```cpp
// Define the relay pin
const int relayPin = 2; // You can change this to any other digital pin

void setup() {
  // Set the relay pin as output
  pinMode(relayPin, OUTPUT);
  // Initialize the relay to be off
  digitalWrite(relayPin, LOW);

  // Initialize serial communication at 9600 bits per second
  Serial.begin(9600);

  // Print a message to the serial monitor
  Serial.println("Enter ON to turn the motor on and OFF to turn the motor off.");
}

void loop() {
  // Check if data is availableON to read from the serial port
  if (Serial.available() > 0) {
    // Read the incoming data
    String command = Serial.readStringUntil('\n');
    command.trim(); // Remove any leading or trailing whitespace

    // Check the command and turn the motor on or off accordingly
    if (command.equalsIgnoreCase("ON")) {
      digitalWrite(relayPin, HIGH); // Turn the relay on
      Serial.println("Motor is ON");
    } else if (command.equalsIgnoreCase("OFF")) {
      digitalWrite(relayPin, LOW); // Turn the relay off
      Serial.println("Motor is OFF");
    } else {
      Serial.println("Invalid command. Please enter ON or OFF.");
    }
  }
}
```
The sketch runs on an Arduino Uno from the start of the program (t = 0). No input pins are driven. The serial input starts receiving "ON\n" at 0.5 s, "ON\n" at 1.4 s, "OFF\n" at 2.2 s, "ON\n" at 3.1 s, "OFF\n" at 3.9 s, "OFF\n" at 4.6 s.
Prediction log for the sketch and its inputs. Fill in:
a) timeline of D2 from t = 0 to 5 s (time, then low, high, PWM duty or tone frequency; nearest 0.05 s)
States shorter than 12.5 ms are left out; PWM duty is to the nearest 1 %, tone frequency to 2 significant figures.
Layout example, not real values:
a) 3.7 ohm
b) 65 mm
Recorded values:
a) 0 s low; 0.5 s high; 2.2 s low; 3.1 s high; 3.9 s low
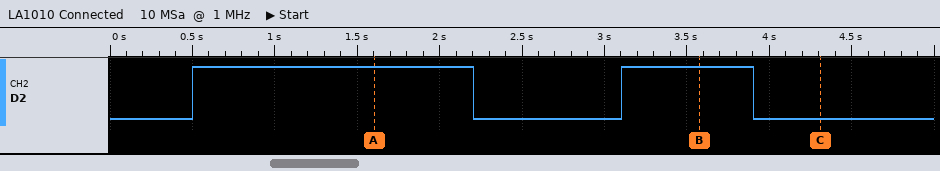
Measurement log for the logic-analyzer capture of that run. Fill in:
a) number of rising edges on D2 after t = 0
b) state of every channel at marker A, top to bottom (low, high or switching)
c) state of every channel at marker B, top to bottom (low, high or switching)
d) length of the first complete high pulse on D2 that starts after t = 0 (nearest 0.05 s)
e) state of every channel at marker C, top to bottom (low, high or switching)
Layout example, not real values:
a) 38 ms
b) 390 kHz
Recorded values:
a) 2
b) D2 high
c) D2 high
d) 1.70 s
e) D2 low
